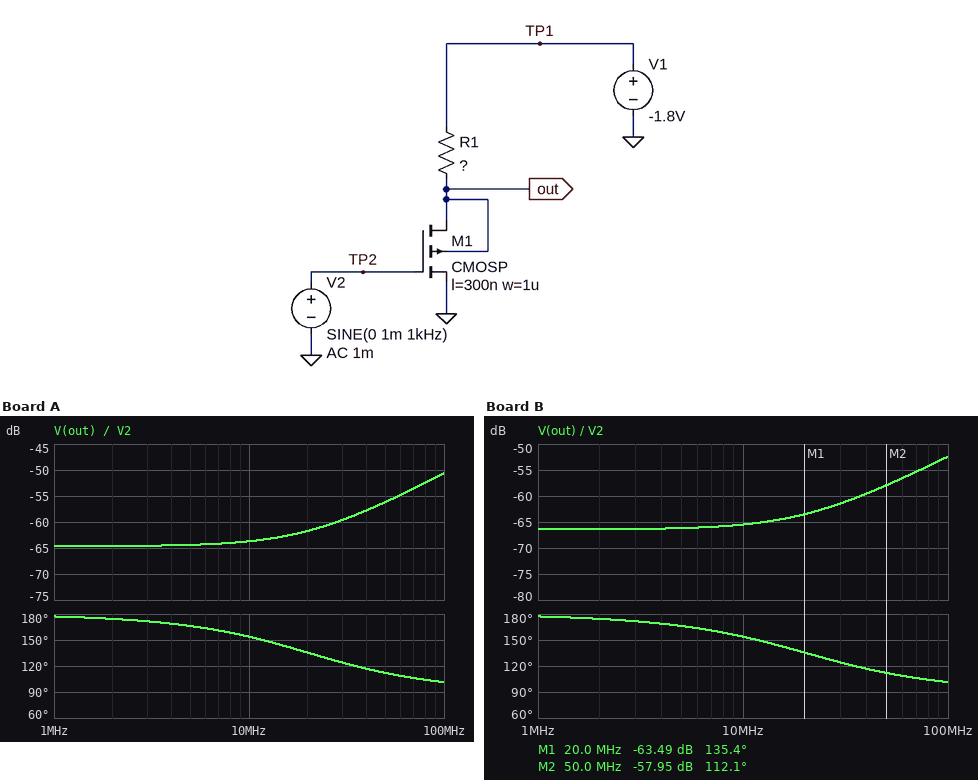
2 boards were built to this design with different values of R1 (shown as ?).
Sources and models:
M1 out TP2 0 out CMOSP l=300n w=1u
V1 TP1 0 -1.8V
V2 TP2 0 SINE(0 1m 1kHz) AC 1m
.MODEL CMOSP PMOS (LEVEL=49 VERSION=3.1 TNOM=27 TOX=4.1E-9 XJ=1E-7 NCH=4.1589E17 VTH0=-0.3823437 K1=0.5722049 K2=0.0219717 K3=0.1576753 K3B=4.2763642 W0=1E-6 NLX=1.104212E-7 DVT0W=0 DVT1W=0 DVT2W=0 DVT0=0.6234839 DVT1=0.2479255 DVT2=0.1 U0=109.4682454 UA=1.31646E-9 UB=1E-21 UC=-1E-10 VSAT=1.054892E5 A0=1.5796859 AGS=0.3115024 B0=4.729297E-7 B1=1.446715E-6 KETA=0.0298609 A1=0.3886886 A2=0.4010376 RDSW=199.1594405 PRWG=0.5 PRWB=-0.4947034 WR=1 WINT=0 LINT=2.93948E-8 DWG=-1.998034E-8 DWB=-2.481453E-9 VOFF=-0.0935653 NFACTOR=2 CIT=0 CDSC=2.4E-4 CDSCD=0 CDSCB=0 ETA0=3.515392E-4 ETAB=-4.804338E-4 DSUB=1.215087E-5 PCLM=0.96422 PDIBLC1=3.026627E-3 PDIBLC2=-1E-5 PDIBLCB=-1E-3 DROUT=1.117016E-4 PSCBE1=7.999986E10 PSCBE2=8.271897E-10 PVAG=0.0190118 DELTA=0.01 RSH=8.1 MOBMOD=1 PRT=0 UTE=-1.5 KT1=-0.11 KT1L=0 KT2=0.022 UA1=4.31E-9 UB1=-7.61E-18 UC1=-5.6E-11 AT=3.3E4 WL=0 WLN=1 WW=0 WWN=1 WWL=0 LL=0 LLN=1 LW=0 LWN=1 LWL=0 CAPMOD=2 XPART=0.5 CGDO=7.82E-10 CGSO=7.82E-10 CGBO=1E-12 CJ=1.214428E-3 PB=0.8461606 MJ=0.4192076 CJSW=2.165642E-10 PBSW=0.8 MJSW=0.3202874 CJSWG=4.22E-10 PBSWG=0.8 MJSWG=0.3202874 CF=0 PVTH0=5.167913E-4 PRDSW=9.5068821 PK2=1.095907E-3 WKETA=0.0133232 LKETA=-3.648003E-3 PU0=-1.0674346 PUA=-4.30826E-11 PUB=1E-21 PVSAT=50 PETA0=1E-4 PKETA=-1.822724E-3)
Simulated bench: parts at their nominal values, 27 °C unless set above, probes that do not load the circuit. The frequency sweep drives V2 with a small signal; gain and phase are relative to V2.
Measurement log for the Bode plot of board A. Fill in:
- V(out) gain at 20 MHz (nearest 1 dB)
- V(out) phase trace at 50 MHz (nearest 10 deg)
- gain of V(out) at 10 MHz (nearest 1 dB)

-62 dB
110 deg
-64 dB
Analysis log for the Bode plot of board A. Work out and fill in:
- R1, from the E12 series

2.7 kΩ
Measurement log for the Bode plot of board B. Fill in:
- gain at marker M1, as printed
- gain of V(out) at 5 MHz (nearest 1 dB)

-63.49 dB
-66 dB
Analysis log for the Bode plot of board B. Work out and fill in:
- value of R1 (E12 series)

2.2 kΩ
